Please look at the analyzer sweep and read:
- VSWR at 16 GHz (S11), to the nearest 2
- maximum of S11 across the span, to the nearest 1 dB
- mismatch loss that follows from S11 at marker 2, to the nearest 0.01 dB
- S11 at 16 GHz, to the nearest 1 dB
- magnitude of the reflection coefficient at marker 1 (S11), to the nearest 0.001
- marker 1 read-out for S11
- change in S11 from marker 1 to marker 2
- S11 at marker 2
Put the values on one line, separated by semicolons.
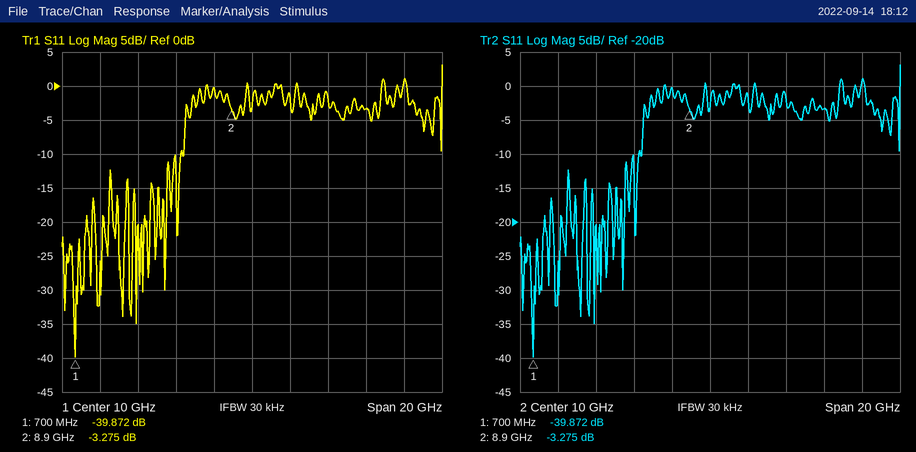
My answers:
6; 3 dB; 2.76 dB; -3 dB; 0.010; -39.872 dB; 36.597 dB; -3.275 dB
